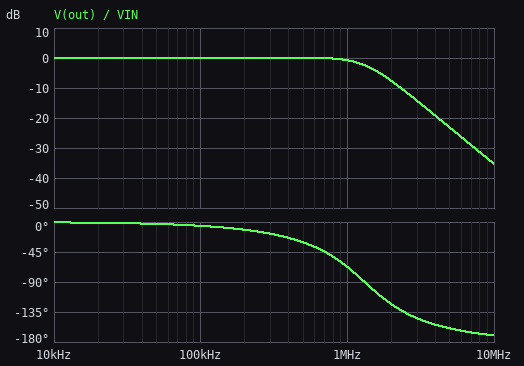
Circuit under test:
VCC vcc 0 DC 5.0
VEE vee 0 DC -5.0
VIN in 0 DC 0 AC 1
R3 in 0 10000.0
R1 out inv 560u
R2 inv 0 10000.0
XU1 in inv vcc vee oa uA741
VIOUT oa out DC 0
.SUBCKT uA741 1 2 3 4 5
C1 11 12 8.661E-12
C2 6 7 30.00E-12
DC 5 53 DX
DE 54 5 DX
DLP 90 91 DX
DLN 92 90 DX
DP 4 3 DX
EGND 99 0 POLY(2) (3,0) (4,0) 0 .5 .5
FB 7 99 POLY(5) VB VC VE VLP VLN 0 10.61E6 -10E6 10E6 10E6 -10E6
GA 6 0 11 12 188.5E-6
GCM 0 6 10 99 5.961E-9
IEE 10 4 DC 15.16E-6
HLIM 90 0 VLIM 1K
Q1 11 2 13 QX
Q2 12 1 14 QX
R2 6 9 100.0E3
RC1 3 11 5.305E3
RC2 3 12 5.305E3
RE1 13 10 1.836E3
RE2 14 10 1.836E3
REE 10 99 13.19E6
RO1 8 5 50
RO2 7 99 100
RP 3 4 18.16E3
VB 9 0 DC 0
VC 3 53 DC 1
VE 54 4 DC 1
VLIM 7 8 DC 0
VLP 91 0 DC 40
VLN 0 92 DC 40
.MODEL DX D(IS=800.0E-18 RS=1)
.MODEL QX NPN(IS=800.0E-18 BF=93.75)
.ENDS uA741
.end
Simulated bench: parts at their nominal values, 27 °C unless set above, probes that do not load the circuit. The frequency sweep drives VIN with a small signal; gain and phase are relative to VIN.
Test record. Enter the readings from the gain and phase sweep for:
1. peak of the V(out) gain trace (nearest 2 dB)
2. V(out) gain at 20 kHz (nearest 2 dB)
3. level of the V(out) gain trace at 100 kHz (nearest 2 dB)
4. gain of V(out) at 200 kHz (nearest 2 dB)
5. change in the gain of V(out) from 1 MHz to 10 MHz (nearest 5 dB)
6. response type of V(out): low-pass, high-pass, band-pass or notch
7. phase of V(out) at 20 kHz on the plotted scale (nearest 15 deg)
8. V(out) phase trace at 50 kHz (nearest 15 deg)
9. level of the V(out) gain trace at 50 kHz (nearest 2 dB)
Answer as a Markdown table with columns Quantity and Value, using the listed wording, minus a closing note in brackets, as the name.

| Quantity | Value |
|---|---|
| peak of the V(out) gain trace | 0 dB |
| V(out) gain at 20 kHz | 0 dB |
| level of the V(out) gain trace at 100 kHz | 0 dB |
| gain of V(out) at 200 kHz | 0 dB |
| change in the gain of V(out) from 1 MHz to 10 MHz | -35 dB |
| response type of V(out): low-pass, high-pass, band-pass or notch | low-pass |
| phase of V(out) at 20 kHz on the plotted scale | 0 deg |
| V(out) phase trace at 50 kHz | 0 deg |
| level of the V(out) gain trace at 50 kHz | 0 dB |
